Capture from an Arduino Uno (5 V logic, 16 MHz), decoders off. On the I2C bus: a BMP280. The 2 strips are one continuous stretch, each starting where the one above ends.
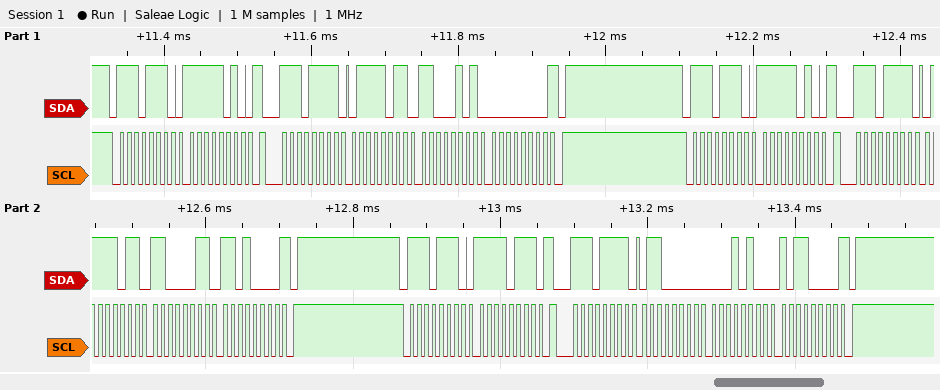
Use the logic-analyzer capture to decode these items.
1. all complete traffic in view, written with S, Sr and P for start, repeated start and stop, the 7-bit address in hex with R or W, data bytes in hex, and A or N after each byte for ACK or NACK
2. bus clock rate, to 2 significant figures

S 77W A FA A Sr 77R A 7B A C5 A 00 N P S 77W A FA A Sr 77R A 7B A C3 A D0 N P S 77W A F7 A Sr 77R A 60 A 14 A B0 N P
100 kHz
